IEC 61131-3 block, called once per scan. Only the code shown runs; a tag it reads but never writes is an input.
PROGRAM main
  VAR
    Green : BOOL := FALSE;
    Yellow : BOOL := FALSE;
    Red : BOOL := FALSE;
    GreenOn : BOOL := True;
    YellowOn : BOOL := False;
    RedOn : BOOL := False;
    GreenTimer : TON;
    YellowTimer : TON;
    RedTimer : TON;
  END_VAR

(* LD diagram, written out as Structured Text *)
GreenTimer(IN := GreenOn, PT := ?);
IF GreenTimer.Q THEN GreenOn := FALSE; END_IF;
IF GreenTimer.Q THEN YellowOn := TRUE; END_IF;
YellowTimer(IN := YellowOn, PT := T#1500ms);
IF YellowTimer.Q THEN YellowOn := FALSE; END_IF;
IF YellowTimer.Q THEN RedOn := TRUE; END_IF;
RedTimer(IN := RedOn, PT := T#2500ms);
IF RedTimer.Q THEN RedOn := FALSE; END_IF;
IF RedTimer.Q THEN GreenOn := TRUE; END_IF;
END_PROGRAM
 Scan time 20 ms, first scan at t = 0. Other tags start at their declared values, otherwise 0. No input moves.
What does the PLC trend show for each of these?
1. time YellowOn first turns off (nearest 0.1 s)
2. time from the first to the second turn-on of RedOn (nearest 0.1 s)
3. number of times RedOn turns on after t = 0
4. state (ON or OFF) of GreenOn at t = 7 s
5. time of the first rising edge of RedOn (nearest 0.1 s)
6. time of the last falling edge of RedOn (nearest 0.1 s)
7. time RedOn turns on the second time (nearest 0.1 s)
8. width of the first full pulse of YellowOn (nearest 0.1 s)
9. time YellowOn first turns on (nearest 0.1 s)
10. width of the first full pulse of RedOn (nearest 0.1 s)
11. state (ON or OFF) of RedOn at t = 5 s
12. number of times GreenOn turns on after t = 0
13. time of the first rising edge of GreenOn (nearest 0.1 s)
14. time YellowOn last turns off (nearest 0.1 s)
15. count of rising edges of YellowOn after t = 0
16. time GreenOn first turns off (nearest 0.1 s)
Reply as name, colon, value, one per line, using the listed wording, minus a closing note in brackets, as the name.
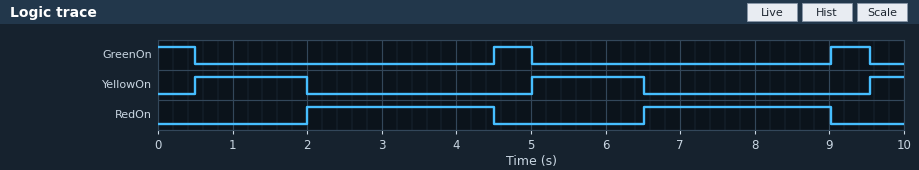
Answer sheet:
time YellowOn first turns off: 2.0 s
time from the first to the second turn-on of RedOn: 4.5 s
number of times RedOn turns on after t = 0: 2
state (ON or OFF) of GreenOn at t = 7 s: OFF
time of the first rising edge of RedOn: 2.0 s
time of the last falling edge of RedOn: 9.0 s
time RedOn turns on the second time: 6.5 s
width of the first full pulse of YellowOn: 1.5 s
time YellowOn first turns on: 0.5 s
width of the first full pulse of RedOn: 2.5 s
state (ON or OFF) of RedOn at t = 5 s: OFF
number of times GreenOn turns on after t = 0: 2
time of the first rising edge of GreenOn: 4.5 s
time YellowOn last turns off: 6.5 s
count of rising edges of YellowOn after t = 0: 3
time GreenOn first turns off: 0.5 s
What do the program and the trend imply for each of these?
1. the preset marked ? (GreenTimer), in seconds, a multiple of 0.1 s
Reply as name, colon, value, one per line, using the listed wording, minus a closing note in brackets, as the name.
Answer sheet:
the preset marked ? (GreenTimer), in seconds, a multiple of 0.1 s: 0.5 s
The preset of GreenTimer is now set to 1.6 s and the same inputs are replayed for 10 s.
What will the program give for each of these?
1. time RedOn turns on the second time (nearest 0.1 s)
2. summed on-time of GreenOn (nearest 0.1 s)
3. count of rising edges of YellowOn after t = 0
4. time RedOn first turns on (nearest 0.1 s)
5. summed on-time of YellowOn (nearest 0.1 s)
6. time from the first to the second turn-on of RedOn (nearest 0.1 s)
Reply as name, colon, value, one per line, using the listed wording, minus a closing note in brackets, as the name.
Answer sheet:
time RedOn turns on the second time: 8.7 s
summed on-time of GreenOn: 3.2 s
count of rising edges of YellowOn after t = 0: 2
time RedOn first turns on: 3.1 s
summed on-time of YellowOn: 3.0 s
time from the first to the second turn-on of RedOn: 5.6 s
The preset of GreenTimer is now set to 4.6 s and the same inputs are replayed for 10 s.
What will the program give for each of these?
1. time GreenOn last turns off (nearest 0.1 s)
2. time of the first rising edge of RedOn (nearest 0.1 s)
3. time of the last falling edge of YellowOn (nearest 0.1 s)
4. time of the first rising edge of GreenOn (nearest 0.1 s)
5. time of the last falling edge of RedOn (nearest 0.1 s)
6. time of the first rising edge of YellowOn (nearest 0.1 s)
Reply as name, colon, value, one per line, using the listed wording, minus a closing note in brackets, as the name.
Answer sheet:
time GreenOn last turns off: 4.6 s
time of the first rising edge of RedOn: 6.1 s
time of the last falling edge of YellowOn: 6.1 s
time of the first rising edge of GreenOn: 8.6 s
time of the last falling edge of RedOn: 8.6 s
time of the first rising edge of YellowOn: 4.6 s
